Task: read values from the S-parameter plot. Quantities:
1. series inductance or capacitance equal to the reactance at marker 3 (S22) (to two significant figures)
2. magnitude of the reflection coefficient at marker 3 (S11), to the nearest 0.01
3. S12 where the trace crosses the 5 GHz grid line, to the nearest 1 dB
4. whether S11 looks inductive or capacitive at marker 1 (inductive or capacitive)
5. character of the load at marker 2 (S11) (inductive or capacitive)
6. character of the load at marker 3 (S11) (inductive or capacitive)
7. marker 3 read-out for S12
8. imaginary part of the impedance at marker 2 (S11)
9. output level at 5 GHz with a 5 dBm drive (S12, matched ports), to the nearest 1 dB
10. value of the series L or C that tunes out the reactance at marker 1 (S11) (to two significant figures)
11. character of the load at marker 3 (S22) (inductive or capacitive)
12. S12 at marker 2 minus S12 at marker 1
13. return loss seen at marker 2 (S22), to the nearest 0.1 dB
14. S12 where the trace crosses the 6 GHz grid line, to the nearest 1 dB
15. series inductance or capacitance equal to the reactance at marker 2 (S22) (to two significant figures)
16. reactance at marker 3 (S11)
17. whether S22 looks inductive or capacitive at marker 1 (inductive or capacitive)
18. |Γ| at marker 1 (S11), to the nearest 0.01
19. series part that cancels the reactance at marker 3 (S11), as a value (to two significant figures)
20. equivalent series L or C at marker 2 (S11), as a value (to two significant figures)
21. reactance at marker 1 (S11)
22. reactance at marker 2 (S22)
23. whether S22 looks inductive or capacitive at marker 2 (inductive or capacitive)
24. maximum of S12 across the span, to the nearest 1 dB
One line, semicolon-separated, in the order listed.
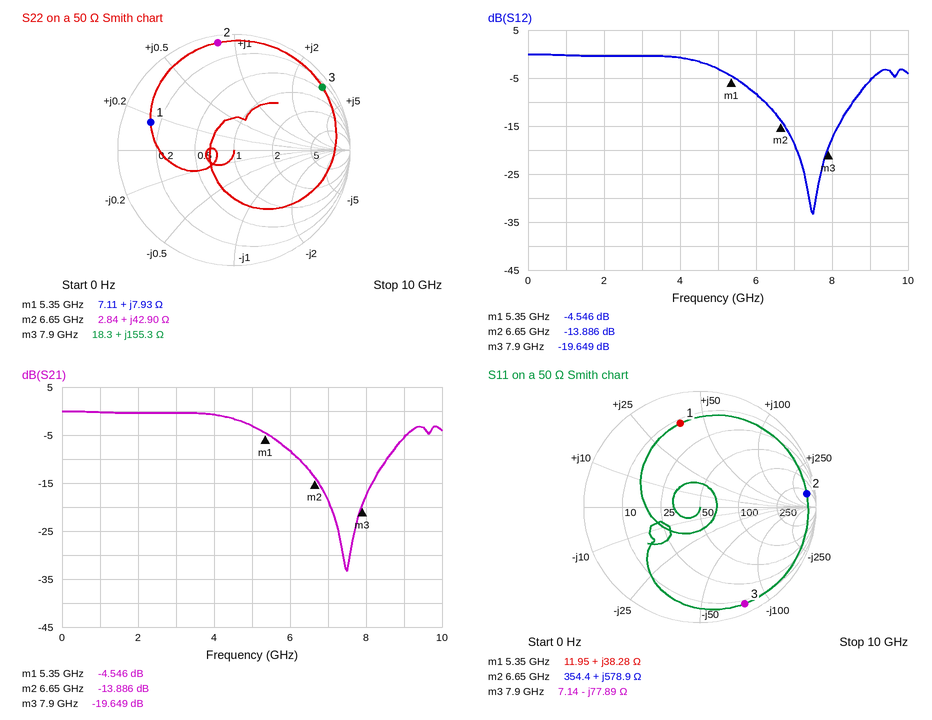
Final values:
3.1 nH; 0.92; -3 dB; inductive; inductive; capacitive; -19.649 dB; +578.9 Ω; 2 dBm; 780 fF; inductive; -9.340 dB; 0.6 dB; -8 dB; 1.0 nH; -77.89 Ω; inductive; 0.74; 1.6 nH; 14 nH; +38.28 Ω; +42.90 Ω; inductive; 0 dB
